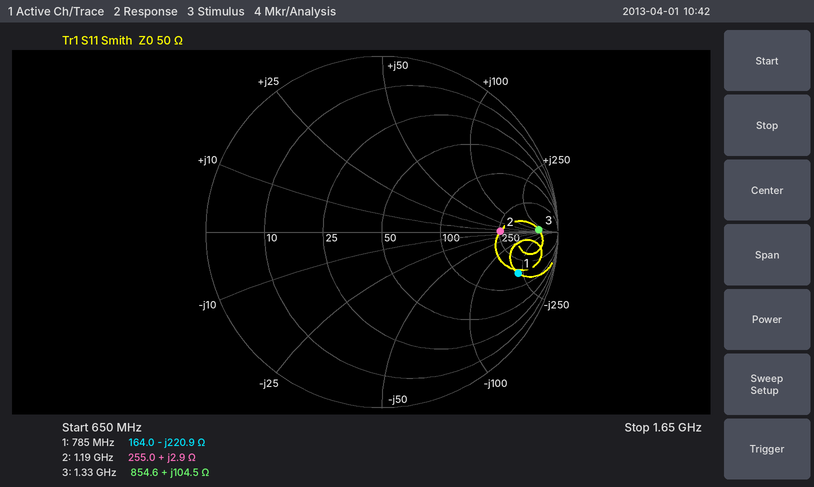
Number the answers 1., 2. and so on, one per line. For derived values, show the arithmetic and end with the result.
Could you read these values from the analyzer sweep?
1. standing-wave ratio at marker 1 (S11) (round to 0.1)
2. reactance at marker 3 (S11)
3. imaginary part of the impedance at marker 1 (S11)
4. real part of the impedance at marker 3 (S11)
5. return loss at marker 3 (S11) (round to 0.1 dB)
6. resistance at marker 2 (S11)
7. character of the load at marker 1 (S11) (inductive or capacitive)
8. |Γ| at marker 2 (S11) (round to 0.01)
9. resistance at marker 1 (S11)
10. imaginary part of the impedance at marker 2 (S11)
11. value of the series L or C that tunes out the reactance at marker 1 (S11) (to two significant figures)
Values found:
1. 9.4
2. +104.5 Ω
3. -220.9 Ω
4. 854.6 Ω
5. 1.0 dB
6. 255.0 Ω
7. capacitive
8. 0.67
9. 164.0 Ω
10. +2.9 Ω
11. L = 220.9 Ω/(2π × 785 MHz) ≈ 45 nH
